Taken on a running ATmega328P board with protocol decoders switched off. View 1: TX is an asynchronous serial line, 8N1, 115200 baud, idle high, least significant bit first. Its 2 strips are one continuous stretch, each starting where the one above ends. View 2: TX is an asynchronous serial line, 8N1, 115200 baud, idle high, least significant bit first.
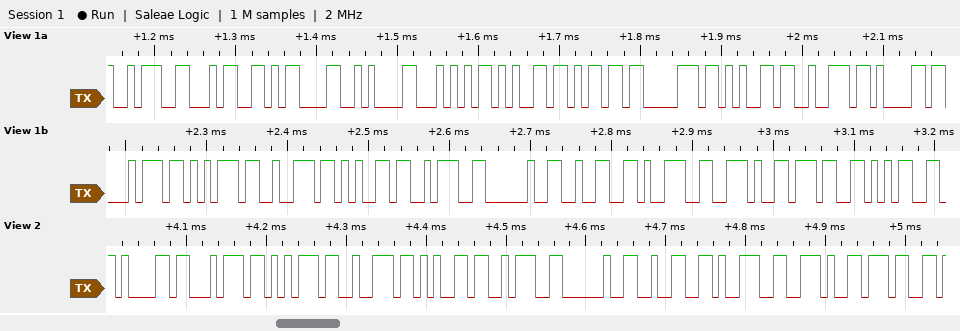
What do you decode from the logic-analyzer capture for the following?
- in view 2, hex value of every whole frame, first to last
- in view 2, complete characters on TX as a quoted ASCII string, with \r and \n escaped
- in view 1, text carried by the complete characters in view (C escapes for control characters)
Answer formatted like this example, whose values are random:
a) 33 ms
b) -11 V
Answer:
a) 0x61 0x74 0x75 0x72 0x65 0x3A 0x20 0x32 0x39 0x2E 0x37
b) "ature: 29.7"
c) ":4\r\nTemperature: 29.75"
